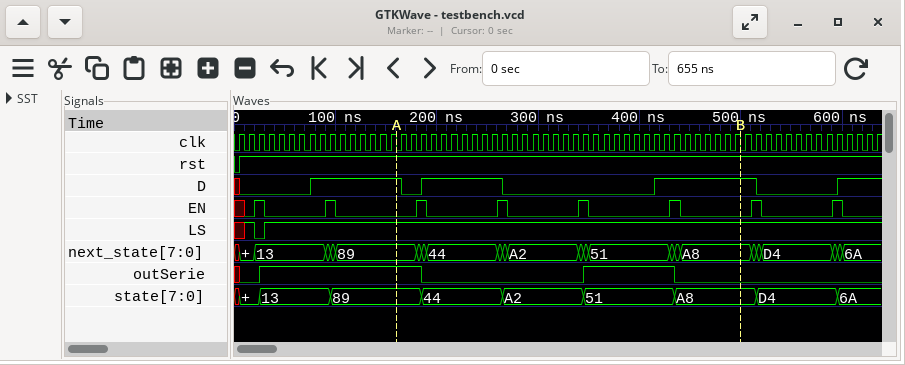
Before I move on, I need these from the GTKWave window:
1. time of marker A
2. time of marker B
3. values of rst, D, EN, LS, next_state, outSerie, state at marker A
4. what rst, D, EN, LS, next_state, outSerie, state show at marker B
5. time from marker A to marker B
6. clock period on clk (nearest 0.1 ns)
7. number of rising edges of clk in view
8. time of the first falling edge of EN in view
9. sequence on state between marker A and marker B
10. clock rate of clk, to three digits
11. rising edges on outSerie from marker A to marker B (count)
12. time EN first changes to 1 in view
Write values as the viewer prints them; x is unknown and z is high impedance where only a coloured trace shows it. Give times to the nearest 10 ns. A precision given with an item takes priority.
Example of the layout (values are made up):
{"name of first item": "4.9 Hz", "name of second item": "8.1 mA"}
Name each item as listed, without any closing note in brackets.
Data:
{"time of marker A": "160 ns", "time of marker B": "500 ns", "values of rst, D, EN, LS, next_state, outSerie, state at marker A": "rst=1, D=1, EN=0, LS=1, next_state=89, outSerie=1, state=89", "what rst, D, EN, LS, next_state, outSerie, state show at marker B": "rst=1, D=1, EN=0, LS=1, next_state=A8, outSerie=0, state=A8", "time from marker A to marker B": "340 ns", "clock period on clk": "10 ns", "number of rising edges of clk in view": "64", "time of the first falling edge of EN in view": "30 ns", "sequence on state between marker A and marker B": "89, 44, A2, 51, A8", "clock rate of clk, to three digits": "100 MHz", "rising edges on outSerie from marker A to marker B": "1", "time EN first changes to 1 in view": "20 ns"}
